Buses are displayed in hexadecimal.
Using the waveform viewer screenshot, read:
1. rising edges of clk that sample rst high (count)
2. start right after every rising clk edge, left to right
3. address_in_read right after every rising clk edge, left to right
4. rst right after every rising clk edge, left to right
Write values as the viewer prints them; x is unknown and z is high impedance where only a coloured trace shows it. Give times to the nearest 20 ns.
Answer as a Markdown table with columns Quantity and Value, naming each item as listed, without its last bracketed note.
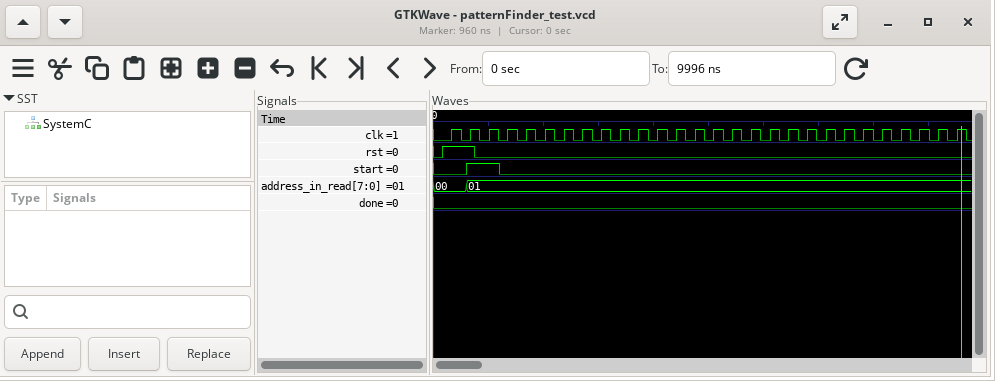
| Quantity | Value |
|---|---|
| rising edges of clk that sample rst high | 2 |
| start right after every rising clk edge, left to right | 0 1 1 0 0 0 0 0 0 0 0 0 0 0 0 0 0 0 0 0 0 0 0 0 0 0 0 0 |
| address_in_read right after every rising clk edge, left to right | 00, 01, 01, 01, 01, 01, 01, 01, 01, 01, 01, 01, 01, 01, 01, 01, 01, 01, 01, 01, 01, 01, 01, 01, 01, 01, 01, 01 |
| rst right after every rising clk edge, left to right | 1 1 0 0 0 0 0 0 0 0 0 0 0 0 0 0 0 0 0 0 0 0 0 0 0 0 0 0 |
